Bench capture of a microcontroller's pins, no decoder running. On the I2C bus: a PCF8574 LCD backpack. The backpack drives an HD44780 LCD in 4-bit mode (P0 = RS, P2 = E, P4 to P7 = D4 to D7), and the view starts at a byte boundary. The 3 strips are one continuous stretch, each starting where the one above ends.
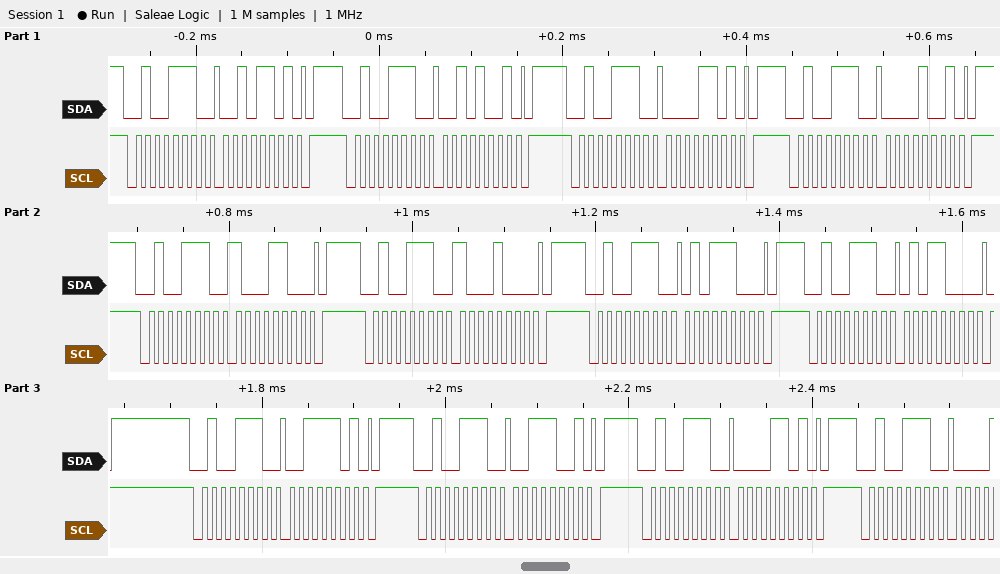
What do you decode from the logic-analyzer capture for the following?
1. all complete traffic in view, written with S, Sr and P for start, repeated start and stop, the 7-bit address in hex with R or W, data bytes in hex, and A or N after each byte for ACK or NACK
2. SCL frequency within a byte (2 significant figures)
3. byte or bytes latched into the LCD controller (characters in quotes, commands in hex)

S 27W A 2D A P S 27W A 29 A P S 27W A 0D A P S 27W A 09 A P S 27W A 8C A P S 27W A 88 A P S 27W A 5C A P S 27W A 58 A P S 27W A 3D A P S 27W A 39 A P S 27W A 0D A P S 27W A
100 kHz
' ' 0x85
